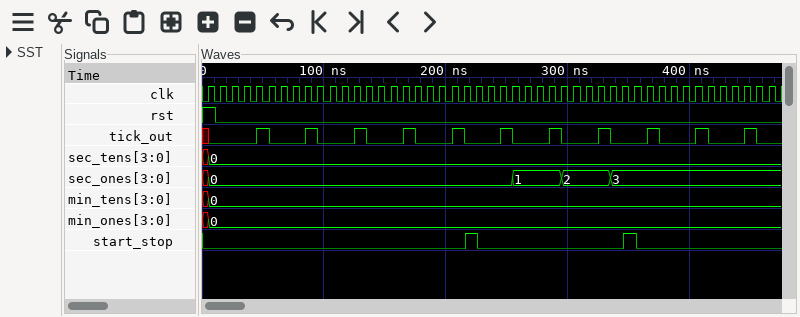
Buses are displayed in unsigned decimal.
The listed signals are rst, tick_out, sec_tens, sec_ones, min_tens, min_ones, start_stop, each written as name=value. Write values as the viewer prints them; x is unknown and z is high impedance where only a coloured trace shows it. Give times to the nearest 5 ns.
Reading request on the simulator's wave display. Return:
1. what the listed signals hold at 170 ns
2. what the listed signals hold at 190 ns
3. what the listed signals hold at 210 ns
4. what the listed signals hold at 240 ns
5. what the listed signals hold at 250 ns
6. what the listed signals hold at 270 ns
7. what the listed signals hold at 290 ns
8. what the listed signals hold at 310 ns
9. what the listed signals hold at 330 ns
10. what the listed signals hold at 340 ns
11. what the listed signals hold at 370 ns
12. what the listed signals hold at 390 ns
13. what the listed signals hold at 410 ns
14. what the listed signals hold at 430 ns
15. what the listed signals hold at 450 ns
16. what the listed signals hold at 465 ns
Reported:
rst=0, tick_out=1, sec_tens=0, sec_ones=0, min_tens=0, min_ones=0, start_stop=0
rst=0, tick_out=0, sec_tens=0, sec_ones=0, min_tens=0, min_ones=0, start_stop=0
rst=0, tick_out=1, sec_tens=0, sec_ones=0, min_tens=0, min_ones=0, start_stop=0
rst=0, tick_out=0, sec_tens=0, sec_ones=0, min_tens=0, min_ones=0, start_stop=0
rst=0, tick_out=1, sec_tens=0, sec_ones=0, min_tens=0, min_ones=0, start_stop=0
rst=0, tick_out=0, sec_tens=0, sec_ones=1, min_tens=0, min_ones=0, start_stop=0
rst=0, tick_out=1, sec_tens=0, sec_ones=1, min_tens=0, min_ones=0, start_stop=0
rst=0, tick_out=0, sec_tens=0, sec_ones=2, min_tens=0, min_ones=0, start_stop=0
rst=0, tick_out=1, sec_tens=0, sec_ones=2, min_tens=0, min_ones=0, start_stop=0
rst=0, tick_out=0, sec_tens=0, sec_ones=3, min_tens=0, min_ones=0, start_stop=0
rst=0, tick_out=1, sec_tens=0, sec_ones=3, min_tens=0, min_ones=0, start_stop=0
rst=0, tick_out=0, sec_tens=0, sec_ones=3, min_tens=0, min_ones=0, start_stop=0
rst=0, tick_out=1, sec_tens=0, sec_ones=3, min_tens=0, min_ones=0, start_stop=0
rst=0, tick_out=0, sec_tens=0, sec_ones=3, min_tens=0, min_ones=0, start_stop=0
rst=0, tick_out=1, sec_tens=0, sec_ones=3, min_tens=0, min_ones=0, start_stop=0
rst=0, tick_out=0, sec_tens=0, sec_ones=3, min_tens=0, min_ones=0, start_stop=0
